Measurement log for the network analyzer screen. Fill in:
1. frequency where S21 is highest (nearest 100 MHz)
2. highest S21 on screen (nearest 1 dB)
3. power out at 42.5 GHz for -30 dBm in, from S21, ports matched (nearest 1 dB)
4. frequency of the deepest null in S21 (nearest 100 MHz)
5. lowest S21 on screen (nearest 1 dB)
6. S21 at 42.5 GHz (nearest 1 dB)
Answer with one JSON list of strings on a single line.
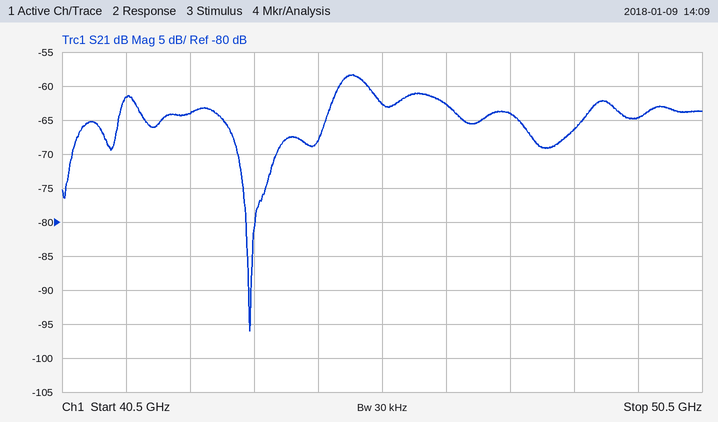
["45.0 GHz", "-58 dB", "-94 dBm", "43.4 GHz", "-96 dB", "-64 dB"]
